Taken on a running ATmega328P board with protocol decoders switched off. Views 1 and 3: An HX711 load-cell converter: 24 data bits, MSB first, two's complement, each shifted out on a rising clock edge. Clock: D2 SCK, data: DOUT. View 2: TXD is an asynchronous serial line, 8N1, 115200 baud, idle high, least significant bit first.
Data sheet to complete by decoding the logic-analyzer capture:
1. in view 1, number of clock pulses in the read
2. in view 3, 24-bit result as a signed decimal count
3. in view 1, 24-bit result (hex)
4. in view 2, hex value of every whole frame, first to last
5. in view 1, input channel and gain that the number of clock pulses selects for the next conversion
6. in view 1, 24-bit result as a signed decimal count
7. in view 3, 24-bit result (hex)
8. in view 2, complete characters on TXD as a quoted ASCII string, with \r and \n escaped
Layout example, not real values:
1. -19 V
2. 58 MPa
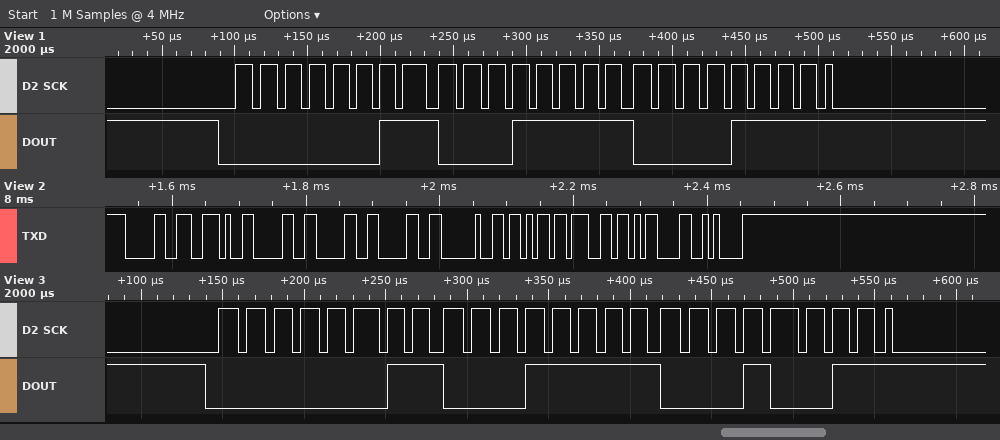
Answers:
1. 25
2. 204563
3. 0x031F0F
4. 0x30 0x2E 0x30 0x30 0x30 0x20 0x6B 0x67 0x0D 0x0A
5. channel A, gain 128
6. 204559
7. 0x031F13
8. "0.000 kg\r\n"
